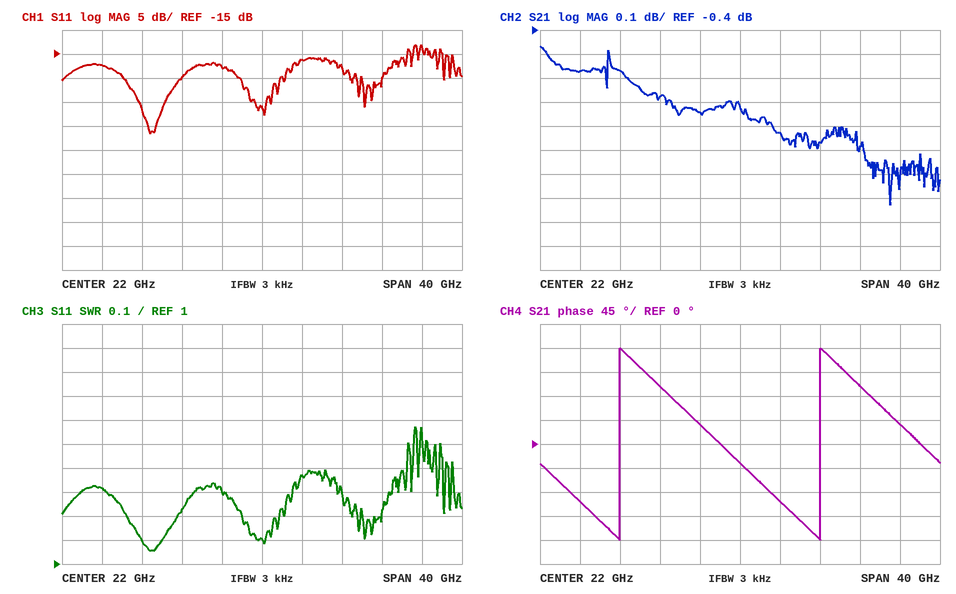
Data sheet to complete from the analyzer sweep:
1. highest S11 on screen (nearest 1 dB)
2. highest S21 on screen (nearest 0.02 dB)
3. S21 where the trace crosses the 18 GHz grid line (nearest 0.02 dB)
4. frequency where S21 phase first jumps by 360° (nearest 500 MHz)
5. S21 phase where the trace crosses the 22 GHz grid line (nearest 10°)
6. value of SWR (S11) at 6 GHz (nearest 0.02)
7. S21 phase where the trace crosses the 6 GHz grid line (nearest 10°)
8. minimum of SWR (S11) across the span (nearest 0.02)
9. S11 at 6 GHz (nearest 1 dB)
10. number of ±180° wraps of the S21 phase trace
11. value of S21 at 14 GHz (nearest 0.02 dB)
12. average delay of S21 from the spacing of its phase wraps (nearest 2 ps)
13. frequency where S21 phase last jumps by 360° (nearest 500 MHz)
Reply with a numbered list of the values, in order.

1. -13 dB
2. -0.46 dB
3. -0.74 dB
4. 10.0 GHz
5. -40°
6. 1.32
7. -110°
8. 1.06
9. -17 dB
10. 2
11. -0.68 dB
12. 50 ps
13. 30.0 GHz
